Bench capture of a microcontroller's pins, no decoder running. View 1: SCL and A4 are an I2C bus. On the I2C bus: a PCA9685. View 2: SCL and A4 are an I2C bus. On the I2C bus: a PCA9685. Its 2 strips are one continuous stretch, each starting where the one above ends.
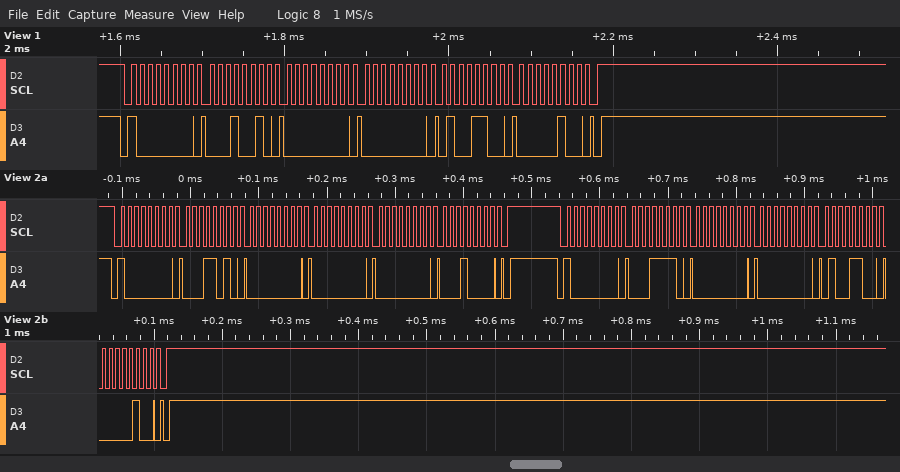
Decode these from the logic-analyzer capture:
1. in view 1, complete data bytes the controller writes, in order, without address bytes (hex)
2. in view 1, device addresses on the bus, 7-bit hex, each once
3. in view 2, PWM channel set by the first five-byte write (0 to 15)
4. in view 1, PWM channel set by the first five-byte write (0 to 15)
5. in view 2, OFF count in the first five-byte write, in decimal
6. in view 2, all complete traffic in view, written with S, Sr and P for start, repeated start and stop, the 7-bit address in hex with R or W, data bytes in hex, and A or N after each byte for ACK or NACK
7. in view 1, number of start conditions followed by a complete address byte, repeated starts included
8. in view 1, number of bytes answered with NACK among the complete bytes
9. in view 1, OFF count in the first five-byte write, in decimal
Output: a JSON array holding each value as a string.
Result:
["12 00 00 4C 04", "0x40", "5", "3", "4096", "S 40W A 1A A 00 A 00 A 00 A 10 A P S 40W A 1E A 00 A 00 A 4C A 04 A P", "1", "0", "1100"]
